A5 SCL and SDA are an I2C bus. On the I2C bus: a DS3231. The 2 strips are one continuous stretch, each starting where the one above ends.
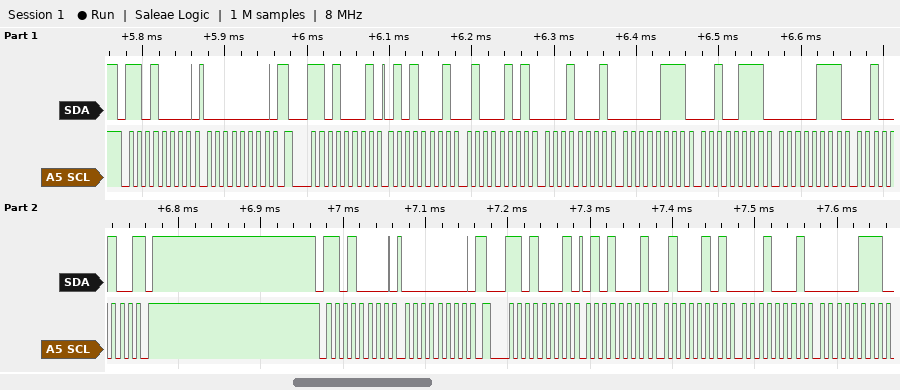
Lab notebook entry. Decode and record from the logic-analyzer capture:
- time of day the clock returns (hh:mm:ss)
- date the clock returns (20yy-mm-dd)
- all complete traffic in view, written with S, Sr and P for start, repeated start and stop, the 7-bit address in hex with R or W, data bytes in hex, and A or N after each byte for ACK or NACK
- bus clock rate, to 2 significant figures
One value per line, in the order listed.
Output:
11:45:51
2024-07-27
S 68W A 00 A Sr 68R A 51 A 45 A 11 A 07 A 27 A 07 A 24 N P S 68W A 00 A Sr 68R A 51 A 45 A 11 A 07 A
100 kHz
